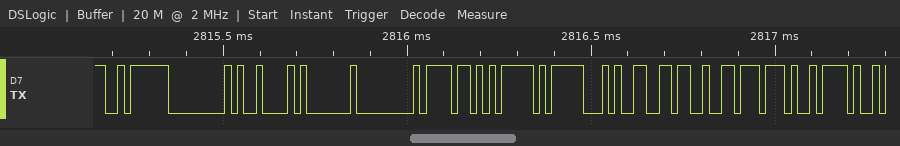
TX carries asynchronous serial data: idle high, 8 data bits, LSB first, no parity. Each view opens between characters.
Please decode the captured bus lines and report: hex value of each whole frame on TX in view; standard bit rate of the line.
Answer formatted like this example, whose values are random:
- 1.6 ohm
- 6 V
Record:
- FA, 00, 09, 01, 00, 6F, 7D, 1F, 99, 93, 77, 7A
- 57600 baud
